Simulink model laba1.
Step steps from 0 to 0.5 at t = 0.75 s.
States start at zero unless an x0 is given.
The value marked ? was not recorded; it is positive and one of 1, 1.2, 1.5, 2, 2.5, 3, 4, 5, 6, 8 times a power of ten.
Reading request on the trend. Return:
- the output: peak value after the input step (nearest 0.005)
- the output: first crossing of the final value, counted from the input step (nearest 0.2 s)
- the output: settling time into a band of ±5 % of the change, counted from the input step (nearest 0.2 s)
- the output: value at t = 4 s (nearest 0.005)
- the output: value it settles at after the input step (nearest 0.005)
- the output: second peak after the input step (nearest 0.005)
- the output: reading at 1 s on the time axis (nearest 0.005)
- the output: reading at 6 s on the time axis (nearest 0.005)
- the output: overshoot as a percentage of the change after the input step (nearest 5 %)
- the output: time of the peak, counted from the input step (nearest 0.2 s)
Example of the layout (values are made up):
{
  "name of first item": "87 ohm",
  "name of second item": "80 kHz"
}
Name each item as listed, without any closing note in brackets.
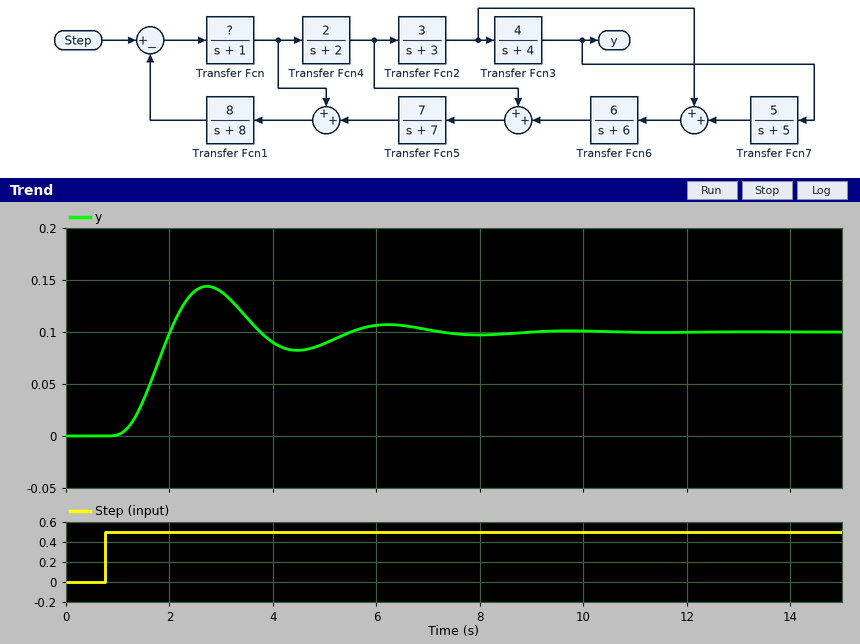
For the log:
{
  "the output: peak value after the input step": "0.145",
  "the output: first crossing of the final value, counted from the input step": "1.2 s",
  "the output: settling time into a band of ±5 % of the change, counted from the input step": "6.0 s",
  "the output: value at t = 4 s": "0.090",
  "the output: value it settles at after the input step": "0.100",
  "the output: second peak after the input step": "0.105",
  "the output: reading at 1 s on the time axis": "0.000",
  "the output: reading at 6 s on the time axis": "0.105",
  "the output: overshoot as a percentage of the change after the input step": "45 %",
  "the output: time of the peak, counted from the input step": "2.0 s"
}
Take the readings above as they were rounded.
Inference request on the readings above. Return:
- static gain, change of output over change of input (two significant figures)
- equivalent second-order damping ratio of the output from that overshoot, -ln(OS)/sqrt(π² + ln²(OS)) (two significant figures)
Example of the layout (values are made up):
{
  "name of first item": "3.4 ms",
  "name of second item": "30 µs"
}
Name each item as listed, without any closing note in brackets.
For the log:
{
  "static gain, change of output over change of input": "0.20",
  "equivalent second-order damping ratio of the output from that overshoot, -ln(OS)/sqrt(π² + ln²(OS))": "0.25"
}
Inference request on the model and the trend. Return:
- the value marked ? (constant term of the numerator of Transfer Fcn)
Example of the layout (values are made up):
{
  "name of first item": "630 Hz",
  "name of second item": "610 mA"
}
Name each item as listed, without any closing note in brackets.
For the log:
{
  "the value marked ?": "1"
}
